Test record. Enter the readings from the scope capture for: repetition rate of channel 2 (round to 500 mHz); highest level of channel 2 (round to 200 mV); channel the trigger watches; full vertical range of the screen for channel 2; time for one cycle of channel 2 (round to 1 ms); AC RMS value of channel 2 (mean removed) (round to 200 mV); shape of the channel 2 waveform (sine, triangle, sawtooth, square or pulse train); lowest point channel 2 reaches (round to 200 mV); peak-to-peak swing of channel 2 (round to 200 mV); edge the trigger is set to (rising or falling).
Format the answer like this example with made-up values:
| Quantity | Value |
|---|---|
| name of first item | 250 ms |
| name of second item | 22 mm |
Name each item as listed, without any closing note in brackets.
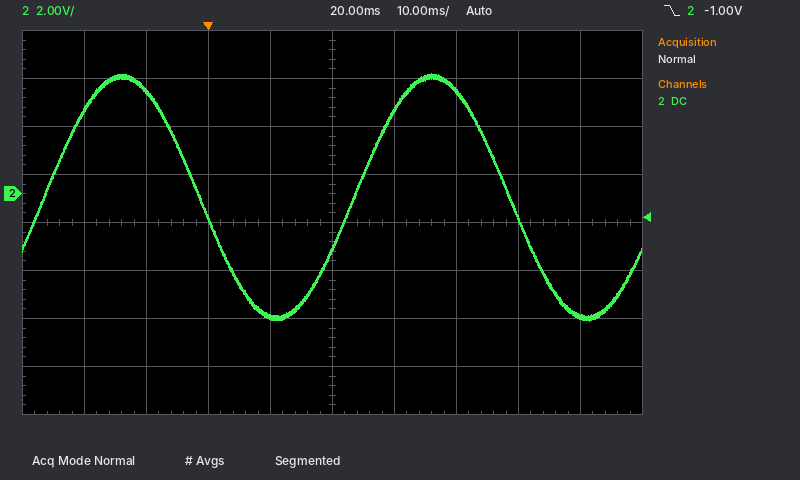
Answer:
| Quantity | Value |
|---|---|
| repetition rate of channel 2 | 20.0 Hz |
| highest level of channel 2 | 5.0 V |
| channel the trigger watches | channel 2 |
| full vertical range of the screen for channel 2 | 16 V |
| time for one cycle of channel 2 | 50 ms |
| AC RMS value of channel 2 (mean removed) | 3.6 V |
| shape of the channel 2 waveform | sine |
| lowest point channel 2 reaches | -5.2 V |
| peak-to-peak swing of channel 2 | 10.2 V |
| edge the trigger is set to | falling |
